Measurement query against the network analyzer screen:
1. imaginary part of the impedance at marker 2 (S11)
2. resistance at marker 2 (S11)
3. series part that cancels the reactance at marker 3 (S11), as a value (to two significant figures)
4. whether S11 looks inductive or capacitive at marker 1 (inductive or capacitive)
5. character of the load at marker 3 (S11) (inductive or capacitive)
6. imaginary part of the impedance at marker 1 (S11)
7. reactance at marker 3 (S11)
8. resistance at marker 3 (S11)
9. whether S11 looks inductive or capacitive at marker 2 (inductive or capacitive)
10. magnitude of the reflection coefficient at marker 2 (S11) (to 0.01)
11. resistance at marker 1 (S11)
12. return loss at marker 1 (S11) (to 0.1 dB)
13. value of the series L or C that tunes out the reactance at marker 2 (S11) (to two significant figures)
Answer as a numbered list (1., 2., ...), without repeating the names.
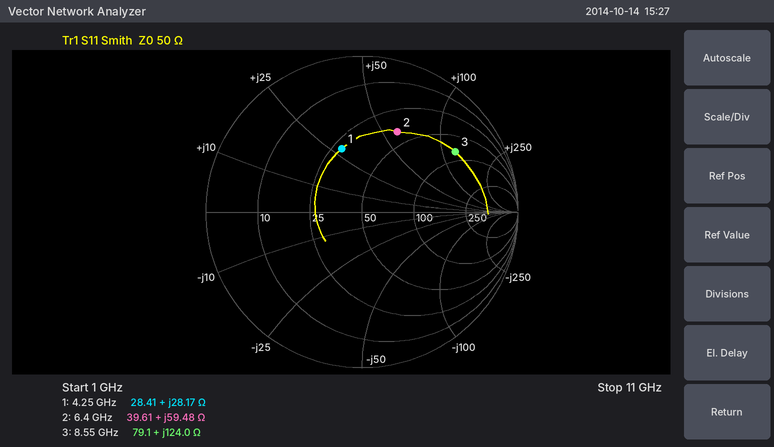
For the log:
1. +59.48 Ω
2. 39.61 Ω
3. 150 fF
4. inductive
5. inductive
6. +28.17 Ω
7. +124.0 Ω
8. 79.1 Ω
9. inductive
10. 0.56
11. 28.41 Ω
12. 7.4 dB
13. 420 fF
